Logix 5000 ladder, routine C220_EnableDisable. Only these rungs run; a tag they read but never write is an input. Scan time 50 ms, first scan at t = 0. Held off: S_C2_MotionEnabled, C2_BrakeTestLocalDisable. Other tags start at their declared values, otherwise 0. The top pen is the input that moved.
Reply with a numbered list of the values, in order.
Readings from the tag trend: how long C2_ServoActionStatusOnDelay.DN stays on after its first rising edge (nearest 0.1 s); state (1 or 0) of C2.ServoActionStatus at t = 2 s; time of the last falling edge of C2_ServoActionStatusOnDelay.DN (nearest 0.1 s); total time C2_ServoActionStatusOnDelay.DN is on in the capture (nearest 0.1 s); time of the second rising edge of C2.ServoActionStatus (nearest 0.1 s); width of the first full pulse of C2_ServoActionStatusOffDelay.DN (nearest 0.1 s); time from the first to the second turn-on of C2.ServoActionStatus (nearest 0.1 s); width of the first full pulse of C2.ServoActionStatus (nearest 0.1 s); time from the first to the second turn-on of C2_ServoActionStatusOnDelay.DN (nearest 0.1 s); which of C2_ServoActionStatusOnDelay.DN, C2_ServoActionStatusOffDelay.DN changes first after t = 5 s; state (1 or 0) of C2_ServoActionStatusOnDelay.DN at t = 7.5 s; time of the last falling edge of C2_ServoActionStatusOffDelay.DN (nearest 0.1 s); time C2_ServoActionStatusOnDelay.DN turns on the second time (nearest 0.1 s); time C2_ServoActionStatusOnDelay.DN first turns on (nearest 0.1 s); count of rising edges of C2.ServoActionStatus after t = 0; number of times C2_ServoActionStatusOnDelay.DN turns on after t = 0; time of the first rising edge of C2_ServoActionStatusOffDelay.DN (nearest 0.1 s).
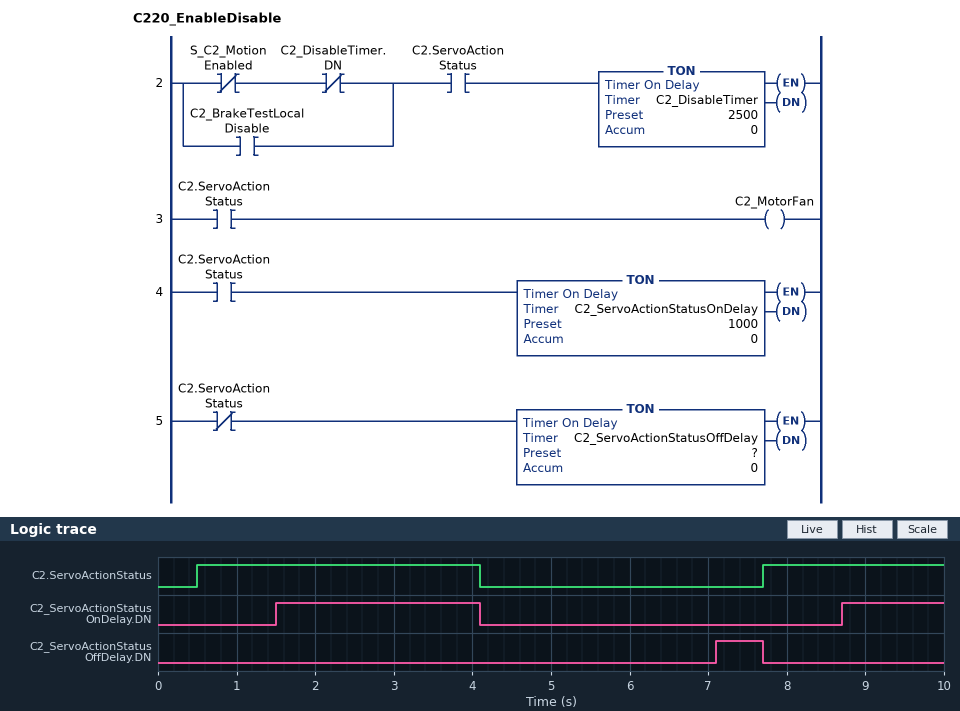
1. 2.6 s
2. 1
3. 4.1 s
4. 3.9 s
5. 7.7 s
6. 0.6 s
7. 7.2 s
8. 3.6 s
9. 7.2 s
10. C2_ServoActionStatusOffDelay.DN
11. 0
12. 7.7 s
13. 8.7 s
14. 1.5 s
15. 2
16. 2
17. 7.1 s
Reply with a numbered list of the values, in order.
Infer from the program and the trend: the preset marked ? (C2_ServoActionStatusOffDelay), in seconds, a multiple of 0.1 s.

1. 3.0 s
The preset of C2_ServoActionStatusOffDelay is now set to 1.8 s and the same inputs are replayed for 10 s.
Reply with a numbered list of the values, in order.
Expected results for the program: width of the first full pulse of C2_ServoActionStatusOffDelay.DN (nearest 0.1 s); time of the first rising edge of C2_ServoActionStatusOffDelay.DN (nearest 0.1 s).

1. 1.8 s
2. 5.9 s
